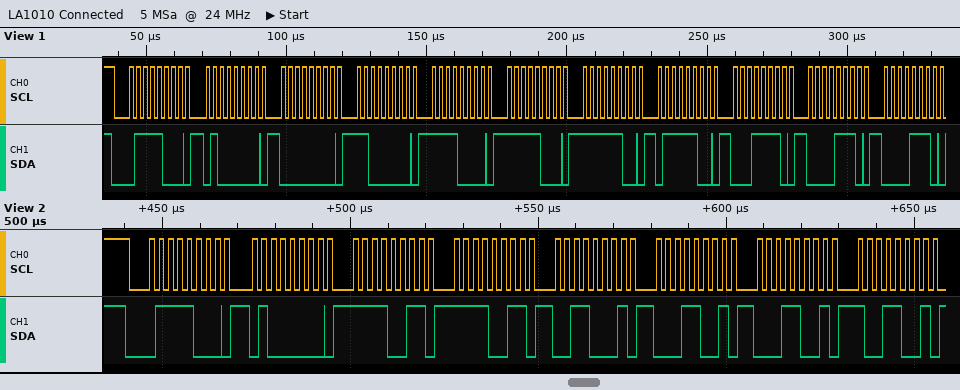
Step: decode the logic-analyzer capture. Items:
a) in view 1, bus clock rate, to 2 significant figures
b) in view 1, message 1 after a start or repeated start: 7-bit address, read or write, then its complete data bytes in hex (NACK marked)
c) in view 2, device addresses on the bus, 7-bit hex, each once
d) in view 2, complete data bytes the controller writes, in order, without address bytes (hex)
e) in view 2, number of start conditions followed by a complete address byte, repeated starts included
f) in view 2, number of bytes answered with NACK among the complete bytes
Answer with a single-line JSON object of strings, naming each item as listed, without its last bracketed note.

{"in view 1, bus clock rate, to 2 significant figures": "400 kHz", "in view 1, message 1 after a start or repeated start: 7-bit address, read or write, then its complete data bytes in hex": "0x3C write: 40 00 C0 F0 F8 FC 7C 1E 0E 0E", "in view 2, device addresses on the bus, 7-bit hex, each once": "0x3C", "in view 2, complete data bytes the controller writes, in order, without address bytes": "40 F3 F3 31 19 19 99", "in view 2, number of start conditions followed by a complete address byte, repeated starts included": "1", "in view 2, number of bytes answered with NACK among the complete bytes": "0"}
